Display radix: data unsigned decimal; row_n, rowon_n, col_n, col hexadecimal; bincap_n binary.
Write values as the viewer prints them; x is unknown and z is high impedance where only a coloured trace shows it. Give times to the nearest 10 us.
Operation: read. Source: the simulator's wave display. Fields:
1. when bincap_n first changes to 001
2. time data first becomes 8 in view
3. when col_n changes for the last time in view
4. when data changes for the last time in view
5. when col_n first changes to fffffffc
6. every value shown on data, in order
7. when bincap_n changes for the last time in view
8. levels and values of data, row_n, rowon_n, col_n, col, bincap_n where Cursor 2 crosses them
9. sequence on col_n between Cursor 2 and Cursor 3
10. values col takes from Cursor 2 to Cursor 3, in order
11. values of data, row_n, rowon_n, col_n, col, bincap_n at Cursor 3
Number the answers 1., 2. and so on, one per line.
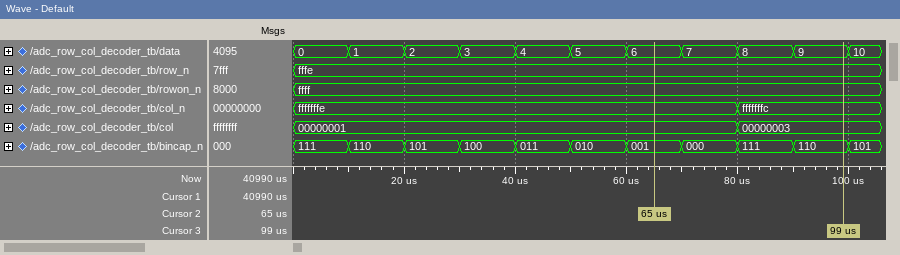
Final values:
1. 60 us
2. 80 us
3. 80 us
4. 100 us
5. 80 us
6. 0, 1, 2, 3, 4, 5, 6, 7, 8, 9, 10
7. 100 us
8. data=6, row_n=fffe, rowon_n=ffff, col_n=fffffffe, col=00000001, bincap_n=001
9. fffffffe, fffffffc
10. 00000001, 00000003
11. data=9, row_n=fffe, rowon_n=ffff, col_n=fffffffc, col=00000003, bincap_n=110
